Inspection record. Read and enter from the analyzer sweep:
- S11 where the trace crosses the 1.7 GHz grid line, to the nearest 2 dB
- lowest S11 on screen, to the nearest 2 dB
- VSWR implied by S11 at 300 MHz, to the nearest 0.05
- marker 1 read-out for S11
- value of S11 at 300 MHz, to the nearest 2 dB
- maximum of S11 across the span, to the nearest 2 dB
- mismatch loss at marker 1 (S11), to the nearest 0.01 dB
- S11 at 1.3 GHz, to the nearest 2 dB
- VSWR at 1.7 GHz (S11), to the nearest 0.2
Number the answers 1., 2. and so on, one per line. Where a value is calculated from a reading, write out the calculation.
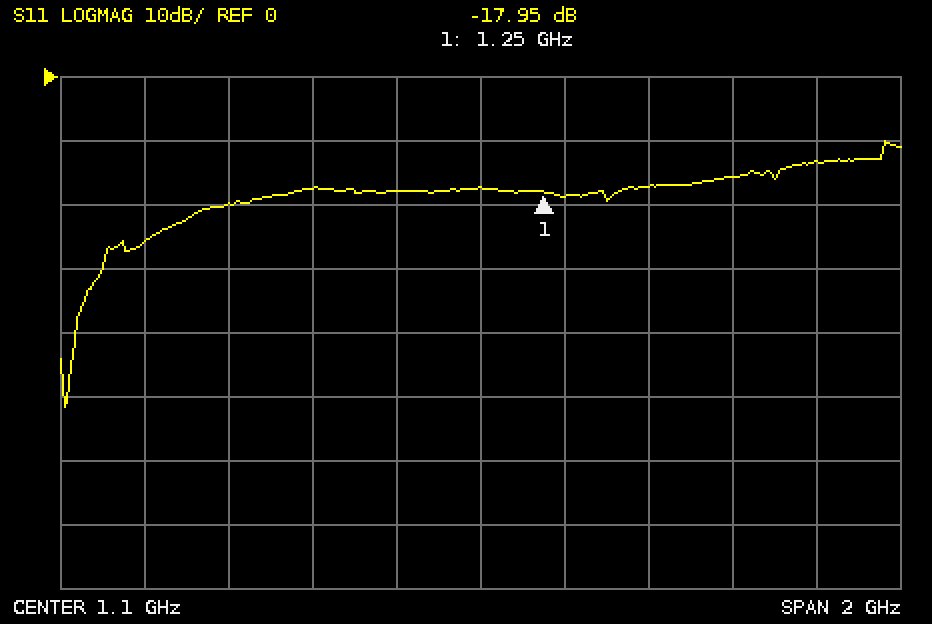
1. -16 dB
2. -52 dB
3. |Γ| = 10^(-26/20) = 0.0501; VSWR = (1 + 0.0501)/(1 − 0.0501) ≈ 1.11, so 1.10 to the nearest 0.05
4. -17.95 dB
5. -26 dB
6. -10 dB
7. −10 log10(1 − 10^(-17.95/10)) ≈ 0.07 dB
8. -18 dB
9. |Γ| = 10^(-16/20) = 0.1585; VSWR = (1 + 0.1585)/(1 − 0.1585) ≈ 1.4
